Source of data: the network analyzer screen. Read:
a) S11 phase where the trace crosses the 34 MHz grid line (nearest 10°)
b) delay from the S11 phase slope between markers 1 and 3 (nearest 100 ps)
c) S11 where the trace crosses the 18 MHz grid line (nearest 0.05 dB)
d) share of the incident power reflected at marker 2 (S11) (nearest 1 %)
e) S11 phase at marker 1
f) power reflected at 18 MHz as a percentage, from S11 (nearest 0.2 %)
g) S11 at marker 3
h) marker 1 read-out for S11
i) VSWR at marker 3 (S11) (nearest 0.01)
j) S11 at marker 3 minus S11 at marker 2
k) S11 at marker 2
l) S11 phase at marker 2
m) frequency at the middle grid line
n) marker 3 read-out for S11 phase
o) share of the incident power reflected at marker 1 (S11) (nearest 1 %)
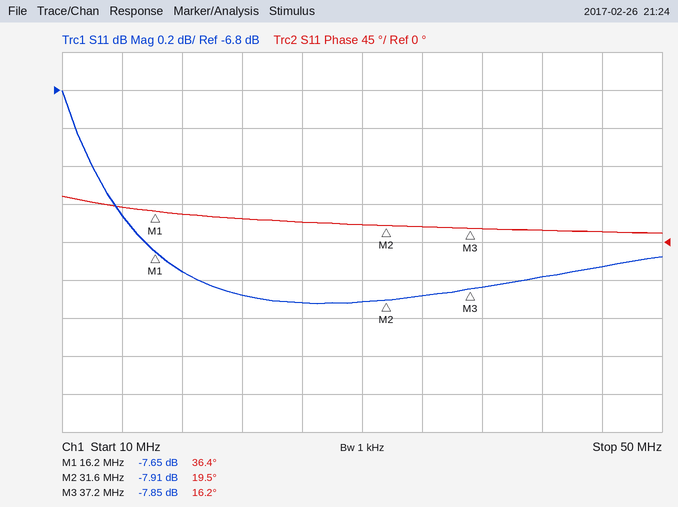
20°
2.7 ns
-7.75 dB
16 %
36.4°
16.8 %
-7.85 dB
-7.65 dB
2.36
0.06 dB
-7.91 dB
19.5°
30 MHz
16.2°
17 %
